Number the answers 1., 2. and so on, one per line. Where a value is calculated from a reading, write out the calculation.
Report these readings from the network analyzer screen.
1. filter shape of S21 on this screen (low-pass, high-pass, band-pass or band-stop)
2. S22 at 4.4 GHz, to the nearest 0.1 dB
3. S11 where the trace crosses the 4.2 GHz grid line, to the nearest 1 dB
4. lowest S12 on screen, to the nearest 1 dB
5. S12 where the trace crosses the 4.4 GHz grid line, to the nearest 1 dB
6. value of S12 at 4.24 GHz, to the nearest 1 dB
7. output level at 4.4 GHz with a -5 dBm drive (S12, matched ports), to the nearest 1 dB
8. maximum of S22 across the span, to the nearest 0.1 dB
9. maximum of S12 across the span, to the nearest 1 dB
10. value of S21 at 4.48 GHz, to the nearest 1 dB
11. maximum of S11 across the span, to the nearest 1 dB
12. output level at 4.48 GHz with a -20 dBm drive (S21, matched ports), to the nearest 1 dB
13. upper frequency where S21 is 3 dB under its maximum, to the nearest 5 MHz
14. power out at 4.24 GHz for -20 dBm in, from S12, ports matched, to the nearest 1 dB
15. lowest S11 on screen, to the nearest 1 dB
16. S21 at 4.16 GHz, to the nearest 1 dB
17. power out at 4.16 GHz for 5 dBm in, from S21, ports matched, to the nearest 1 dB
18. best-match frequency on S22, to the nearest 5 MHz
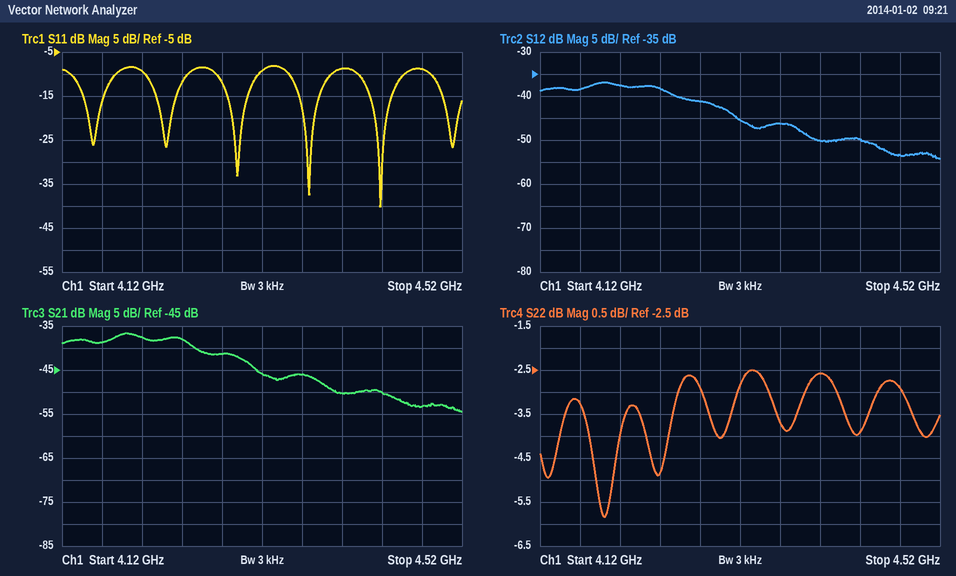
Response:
1. low-pass
2. -2.6 dB
3. -9 dB
4. -54 dB
5. -50 dB
6. -38 dB
7. -5 dBm + (-50 dB) = -55 dBm
8. -2.5 dB
9. -37 dB
10. -53 dB
11. -8 dB
12. -20 dBm + (-53 dB) = -73 dBm
13. 4.250 GHz
14. -20 dBm + (-38 dB) = -58 dBm
15. -40 dB
16. -39 dB
17. 5 dBm + (-39 dB) = -34 dBm
18. 4.185 GHz
